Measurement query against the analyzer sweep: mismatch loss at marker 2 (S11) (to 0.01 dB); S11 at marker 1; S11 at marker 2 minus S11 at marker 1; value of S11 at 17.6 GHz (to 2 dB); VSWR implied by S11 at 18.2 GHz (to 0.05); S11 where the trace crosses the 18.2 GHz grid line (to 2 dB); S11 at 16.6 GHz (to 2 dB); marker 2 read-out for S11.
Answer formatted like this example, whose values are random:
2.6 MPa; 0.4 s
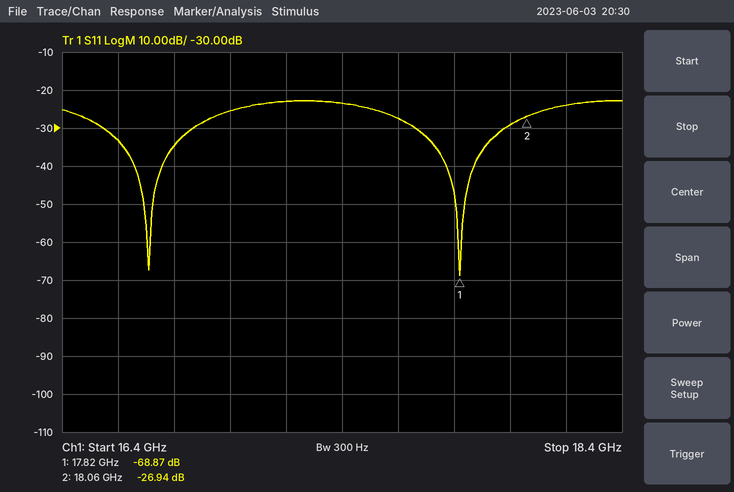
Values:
0.01 dB; -68.87 dB; 41.93 dB; -28 dB; 1.15; -24 dB; -34 dB; -26.94 dB
